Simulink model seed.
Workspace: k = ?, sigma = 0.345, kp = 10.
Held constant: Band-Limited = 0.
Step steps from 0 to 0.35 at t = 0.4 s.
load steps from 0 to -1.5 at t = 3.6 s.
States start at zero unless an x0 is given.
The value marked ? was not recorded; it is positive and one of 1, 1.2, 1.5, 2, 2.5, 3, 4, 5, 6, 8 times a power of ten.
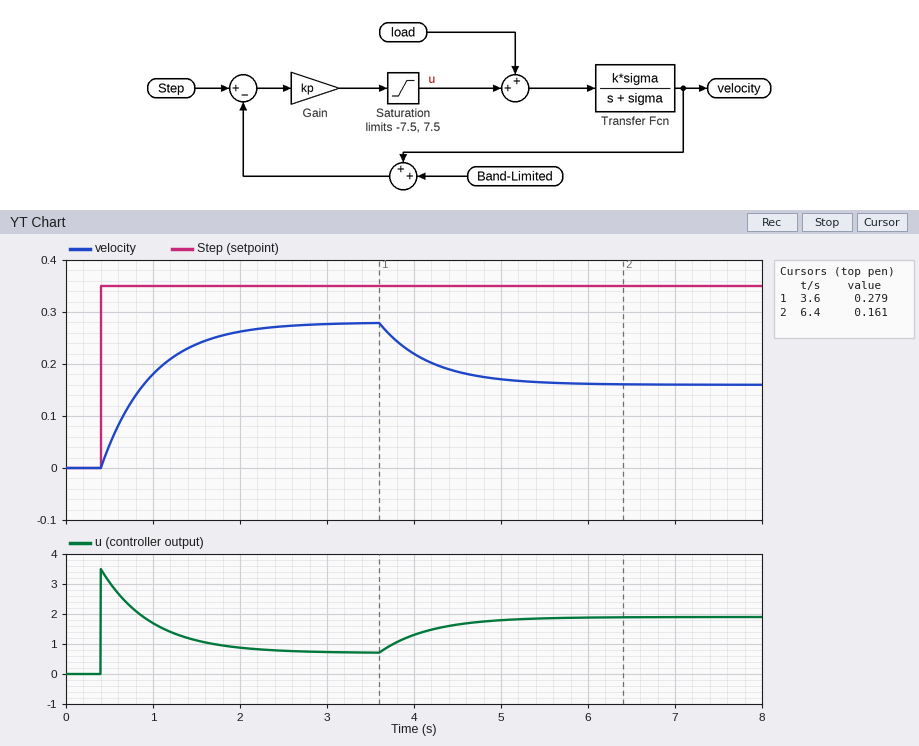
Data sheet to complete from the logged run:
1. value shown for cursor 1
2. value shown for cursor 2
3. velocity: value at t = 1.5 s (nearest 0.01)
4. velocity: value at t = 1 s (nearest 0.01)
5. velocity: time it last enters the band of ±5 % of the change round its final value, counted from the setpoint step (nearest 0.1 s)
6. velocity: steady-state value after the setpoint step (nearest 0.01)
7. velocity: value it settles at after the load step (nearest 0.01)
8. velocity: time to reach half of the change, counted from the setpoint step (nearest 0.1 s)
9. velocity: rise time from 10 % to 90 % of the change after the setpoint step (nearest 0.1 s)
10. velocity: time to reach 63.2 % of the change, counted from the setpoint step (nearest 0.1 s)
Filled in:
0.279
0.161
0.24
0.18
1.7 s
0.28
0.16
0.4 s
1.3 s
0.6 s
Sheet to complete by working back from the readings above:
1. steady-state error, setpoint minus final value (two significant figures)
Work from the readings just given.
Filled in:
0.070
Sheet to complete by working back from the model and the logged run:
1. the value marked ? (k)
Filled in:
0.4
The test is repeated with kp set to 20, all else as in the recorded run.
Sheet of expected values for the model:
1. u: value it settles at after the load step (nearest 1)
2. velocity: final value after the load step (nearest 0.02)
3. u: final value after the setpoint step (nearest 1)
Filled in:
2
0.24
1
